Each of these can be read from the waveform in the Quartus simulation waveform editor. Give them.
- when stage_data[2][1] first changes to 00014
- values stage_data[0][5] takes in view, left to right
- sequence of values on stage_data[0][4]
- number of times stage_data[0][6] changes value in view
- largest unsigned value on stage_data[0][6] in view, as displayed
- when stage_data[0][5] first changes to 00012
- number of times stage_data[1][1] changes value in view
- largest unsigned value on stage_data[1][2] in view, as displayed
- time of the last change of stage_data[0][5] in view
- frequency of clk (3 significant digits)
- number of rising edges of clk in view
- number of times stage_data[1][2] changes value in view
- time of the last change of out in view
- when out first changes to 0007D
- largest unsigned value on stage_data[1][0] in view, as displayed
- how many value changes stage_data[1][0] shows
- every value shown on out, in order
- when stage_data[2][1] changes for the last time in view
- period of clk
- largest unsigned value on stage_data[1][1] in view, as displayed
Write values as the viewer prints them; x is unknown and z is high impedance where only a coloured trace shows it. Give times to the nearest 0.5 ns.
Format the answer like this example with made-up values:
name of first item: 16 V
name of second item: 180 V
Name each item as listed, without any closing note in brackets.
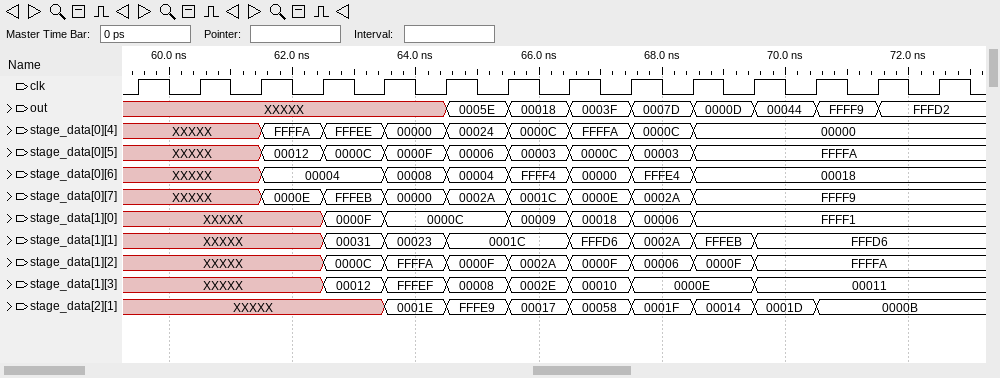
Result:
when stage_data[2][1] first changes to 00014: 68.5 ns
values stage_data[0][5] takes in view, left to right: XXXXX, 00012, 0000C, 0000F, 00006, 00003, 0000C, 00003, FFFFA
sequence of values on stage_data[0][4]: XXXXX, FFFFA, FFFEE, 00000, 00024, 0000C, FFFFA, 0000C, 00000
number of times stage_data[0][6] changes value in view: 7
largest unsigned value on stage_data[0][6] in view, as displayed: FFFF4
when stage_data[0][5] first changes to 00012: 61.5 ns
number of times stage_data[1][1] changes value in view: 7
largest unsigned value on stage_data[1][2] in view, as displayed: FFFFA
time of the last change of stage_data[0][5] in view: 68.5 ns
frequency of clk: 1.00 GHz
number of rising edges of clk in view: 14
number of times stage_data[1][2] changes value in view: 8
time of the last change of out in view: 71.5 ns
when out first changes to 0007D: 67.5 ns
largest unsigned value on stage_data[1][0] in view, as displayed: FFFF1
how many value changes stage_data[1][0] shows: 6
every value shown on out, in order: XXXXX, 0005E, 00018, 0003F, 0007D, 0000D, 00044, FFFF9, FFFD2
when stage_data[2][1] changes for the last time in view: 70.5 ns
period of clk: 1 ns
largest unsigned value on stage_data[1][1] in view, as displayed: FFFEB
